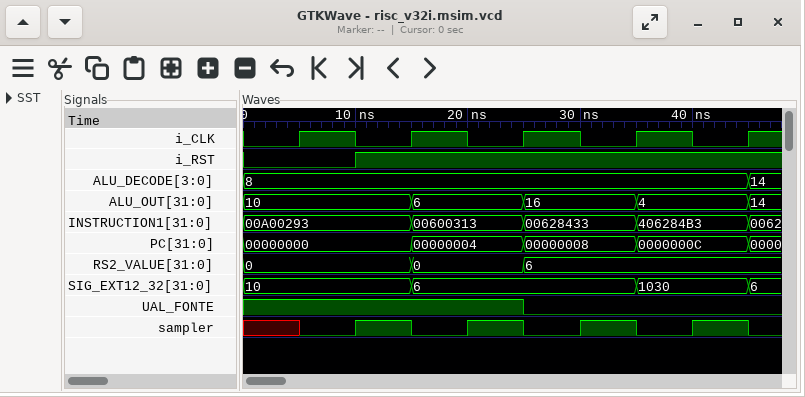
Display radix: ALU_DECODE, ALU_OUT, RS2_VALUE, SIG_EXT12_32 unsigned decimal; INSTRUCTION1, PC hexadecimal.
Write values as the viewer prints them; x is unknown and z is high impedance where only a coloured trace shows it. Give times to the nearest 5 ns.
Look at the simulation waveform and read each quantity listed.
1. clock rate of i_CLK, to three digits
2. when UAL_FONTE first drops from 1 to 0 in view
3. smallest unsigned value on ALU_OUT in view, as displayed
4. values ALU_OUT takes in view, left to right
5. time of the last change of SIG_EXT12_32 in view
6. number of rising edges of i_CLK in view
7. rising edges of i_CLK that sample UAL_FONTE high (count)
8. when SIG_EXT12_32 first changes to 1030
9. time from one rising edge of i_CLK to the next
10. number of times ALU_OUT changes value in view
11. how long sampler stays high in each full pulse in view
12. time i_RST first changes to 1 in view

100 MHz
25 ns
4
10, 6, 16, 4, 14
45 ns
5
3
35 ns
10 ns
4
5 ns, 5 ns, 5 ns, 5 ns
10 ns
